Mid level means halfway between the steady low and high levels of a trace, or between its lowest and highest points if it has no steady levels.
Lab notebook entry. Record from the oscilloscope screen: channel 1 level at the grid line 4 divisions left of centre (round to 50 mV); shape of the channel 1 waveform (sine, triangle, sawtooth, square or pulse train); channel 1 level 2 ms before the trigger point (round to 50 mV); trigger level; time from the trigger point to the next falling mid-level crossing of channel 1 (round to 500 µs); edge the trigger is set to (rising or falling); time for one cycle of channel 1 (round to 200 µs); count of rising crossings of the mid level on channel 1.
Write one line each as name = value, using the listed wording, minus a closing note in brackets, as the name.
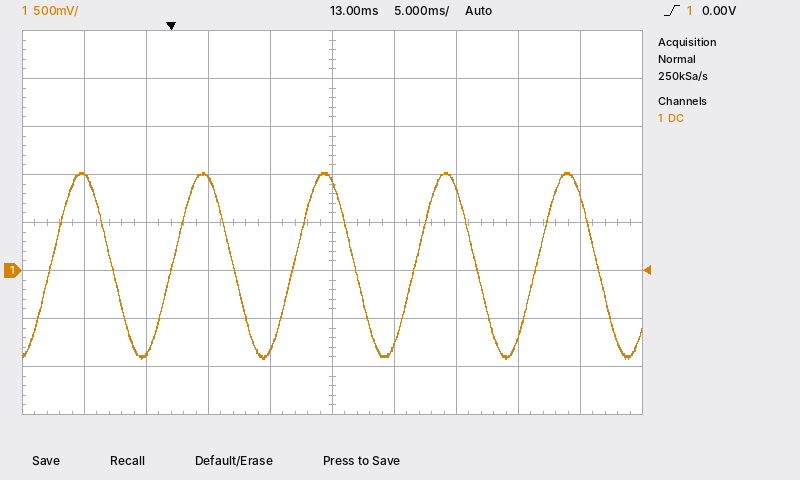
channel 1 level at the grid line 4 divisions left of centre = 1.00 V
shape of the channel 1 waveform = sine
channel 1 level 2 ms before the trigger point = -850 mV
trigger level = 0.00 V
time from the trigger point to the next falling mid-level crossing of channel 1 = 5.0 ms
edge the trigger is set to = rising
time for one cycle of channel 1 = 9.8 ms
count of rising crossings of the mid level on channel 1 = 5
